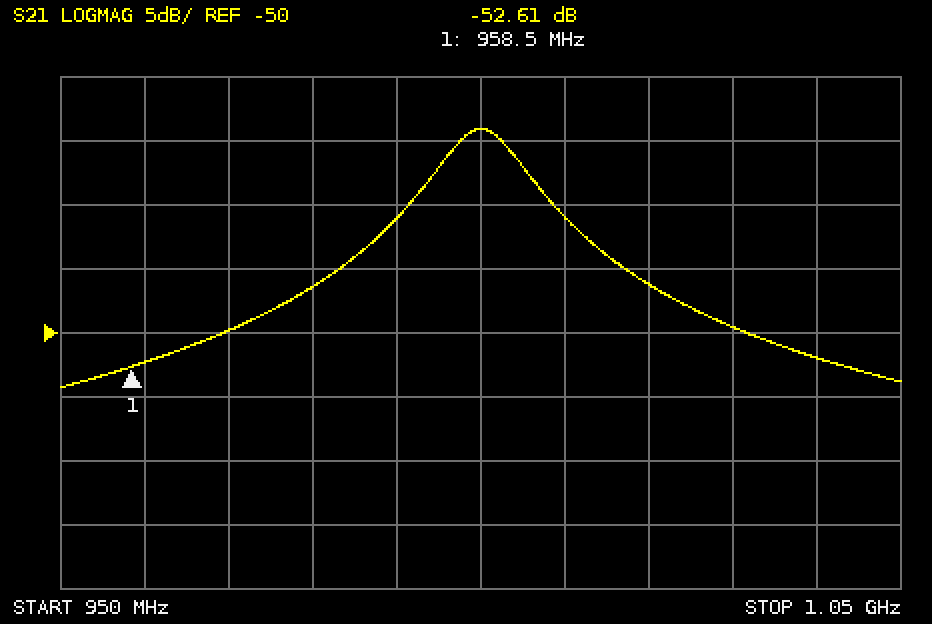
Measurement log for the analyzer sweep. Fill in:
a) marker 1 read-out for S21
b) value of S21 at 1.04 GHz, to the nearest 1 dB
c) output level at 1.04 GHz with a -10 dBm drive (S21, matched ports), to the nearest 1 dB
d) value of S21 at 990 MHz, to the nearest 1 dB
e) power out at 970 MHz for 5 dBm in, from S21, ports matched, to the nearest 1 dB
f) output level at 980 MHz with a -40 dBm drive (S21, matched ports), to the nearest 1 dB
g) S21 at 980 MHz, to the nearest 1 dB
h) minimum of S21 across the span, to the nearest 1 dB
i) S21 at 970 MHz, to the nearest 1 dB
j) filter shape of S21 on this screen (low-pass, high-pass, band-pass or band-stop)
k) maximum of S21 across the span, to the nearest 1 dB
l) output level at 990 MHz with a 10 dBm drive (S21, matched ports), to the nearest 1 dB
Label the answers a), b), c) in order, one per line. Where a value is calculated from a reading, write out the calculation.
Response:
a) -52.61 dB
b) -52 dB
c) -10 dBm + (-52 dB) = -62 dBm
d) -41 dB
e) 5 dBm + (-50 dB) = -45 dBm
f) -40 dBm + (-46 dB) = -86 dBm
g) -46 dB
h) -54 dB
i) -50 dB
j) band-pass
k) -34 dB
l) 10 dBm + (-41 dB) = -31 dBm
